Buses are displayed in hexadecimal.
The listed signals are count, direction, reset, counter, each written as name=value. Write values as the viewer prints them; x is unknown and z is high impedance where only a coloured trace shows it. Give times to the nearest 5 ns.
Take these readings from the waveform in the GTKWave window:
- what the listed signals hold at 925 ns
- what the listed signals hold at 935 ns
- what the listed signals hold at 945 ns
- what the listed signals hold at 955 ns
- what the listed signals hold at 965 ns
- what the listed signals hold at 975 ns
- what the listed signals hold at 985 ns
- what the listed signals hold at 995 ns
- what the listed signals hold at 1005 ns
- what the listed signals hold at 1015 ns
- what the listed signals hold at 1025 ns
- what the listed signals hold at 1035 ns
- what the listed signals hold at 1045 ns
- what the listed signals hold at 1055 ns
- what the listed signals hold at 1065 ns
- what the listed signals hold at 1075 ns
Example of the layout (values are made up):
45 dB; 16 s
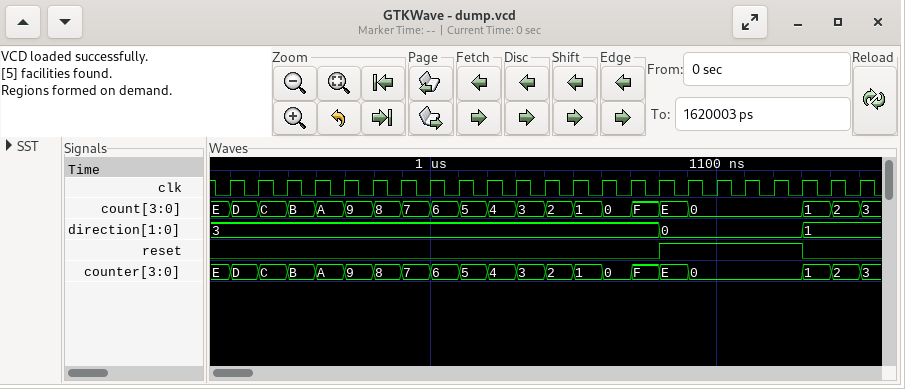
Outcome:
count=E, direction=3, reset=0, counter=E; count=D, direction=3, reset=0, counter=D; count=C, direction=3, reset=0, counter=C; count=B, direction=3, reset=0, counter=B; count=A, direction=3, reset=0, counter=A; count=9, direction=3, reset=0, counter=9; count=8, direction=3, reset=0, counter=8; count=7, direction=3, reset=0, counter=7; count=6, direction=3, reset=0, counter=6; count=5, direction=3, reset=0, counter=5; count=4, direction=3, reset=0, counter=4; count=3, direction=3, reset=0, counter=3; count=2, direction=3, reset=0, counter=2; count=1, direction=3, reset=0, counter=1; count=0, direction=3, reset=0, counter=0; count=F, direction=3, reset=0, counter=F
